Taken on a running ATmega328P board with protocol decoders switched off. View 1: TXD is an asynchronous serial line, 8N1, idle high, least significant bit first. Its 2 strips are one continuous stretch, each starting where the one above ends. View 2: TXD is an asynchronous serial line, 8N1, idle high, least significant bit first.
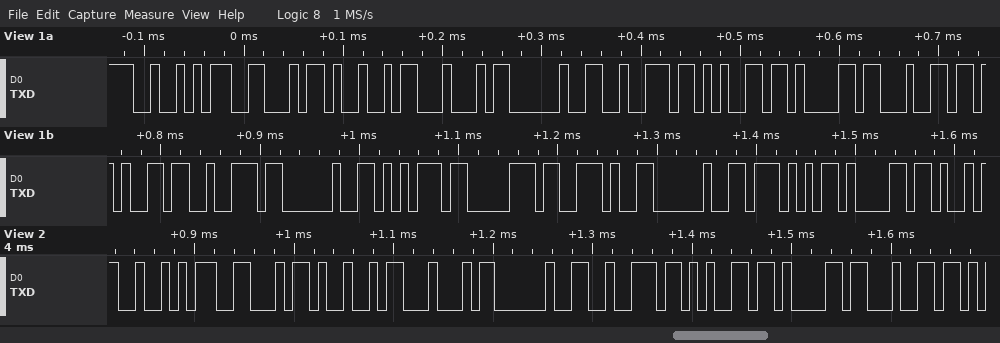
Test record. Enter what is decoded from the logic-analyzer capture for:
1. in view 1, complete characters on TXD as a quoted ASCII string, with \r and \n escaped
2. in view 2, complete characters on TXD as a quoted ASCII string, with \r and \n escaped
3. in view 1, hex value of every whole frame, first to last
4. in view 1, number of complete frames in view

"RFID reader up. Wa"
"RFID read"
52 46 49 44 20 72 65 61 64 65 72 20 75 70 2E 20 57 61
18
